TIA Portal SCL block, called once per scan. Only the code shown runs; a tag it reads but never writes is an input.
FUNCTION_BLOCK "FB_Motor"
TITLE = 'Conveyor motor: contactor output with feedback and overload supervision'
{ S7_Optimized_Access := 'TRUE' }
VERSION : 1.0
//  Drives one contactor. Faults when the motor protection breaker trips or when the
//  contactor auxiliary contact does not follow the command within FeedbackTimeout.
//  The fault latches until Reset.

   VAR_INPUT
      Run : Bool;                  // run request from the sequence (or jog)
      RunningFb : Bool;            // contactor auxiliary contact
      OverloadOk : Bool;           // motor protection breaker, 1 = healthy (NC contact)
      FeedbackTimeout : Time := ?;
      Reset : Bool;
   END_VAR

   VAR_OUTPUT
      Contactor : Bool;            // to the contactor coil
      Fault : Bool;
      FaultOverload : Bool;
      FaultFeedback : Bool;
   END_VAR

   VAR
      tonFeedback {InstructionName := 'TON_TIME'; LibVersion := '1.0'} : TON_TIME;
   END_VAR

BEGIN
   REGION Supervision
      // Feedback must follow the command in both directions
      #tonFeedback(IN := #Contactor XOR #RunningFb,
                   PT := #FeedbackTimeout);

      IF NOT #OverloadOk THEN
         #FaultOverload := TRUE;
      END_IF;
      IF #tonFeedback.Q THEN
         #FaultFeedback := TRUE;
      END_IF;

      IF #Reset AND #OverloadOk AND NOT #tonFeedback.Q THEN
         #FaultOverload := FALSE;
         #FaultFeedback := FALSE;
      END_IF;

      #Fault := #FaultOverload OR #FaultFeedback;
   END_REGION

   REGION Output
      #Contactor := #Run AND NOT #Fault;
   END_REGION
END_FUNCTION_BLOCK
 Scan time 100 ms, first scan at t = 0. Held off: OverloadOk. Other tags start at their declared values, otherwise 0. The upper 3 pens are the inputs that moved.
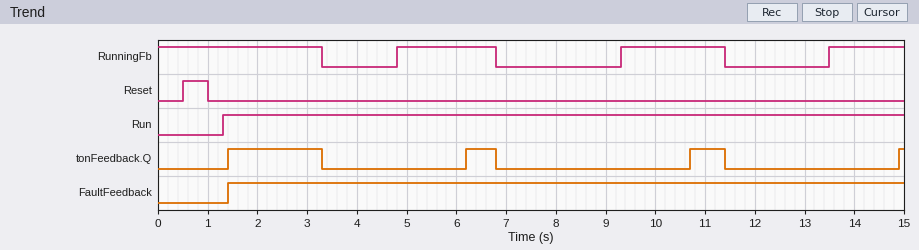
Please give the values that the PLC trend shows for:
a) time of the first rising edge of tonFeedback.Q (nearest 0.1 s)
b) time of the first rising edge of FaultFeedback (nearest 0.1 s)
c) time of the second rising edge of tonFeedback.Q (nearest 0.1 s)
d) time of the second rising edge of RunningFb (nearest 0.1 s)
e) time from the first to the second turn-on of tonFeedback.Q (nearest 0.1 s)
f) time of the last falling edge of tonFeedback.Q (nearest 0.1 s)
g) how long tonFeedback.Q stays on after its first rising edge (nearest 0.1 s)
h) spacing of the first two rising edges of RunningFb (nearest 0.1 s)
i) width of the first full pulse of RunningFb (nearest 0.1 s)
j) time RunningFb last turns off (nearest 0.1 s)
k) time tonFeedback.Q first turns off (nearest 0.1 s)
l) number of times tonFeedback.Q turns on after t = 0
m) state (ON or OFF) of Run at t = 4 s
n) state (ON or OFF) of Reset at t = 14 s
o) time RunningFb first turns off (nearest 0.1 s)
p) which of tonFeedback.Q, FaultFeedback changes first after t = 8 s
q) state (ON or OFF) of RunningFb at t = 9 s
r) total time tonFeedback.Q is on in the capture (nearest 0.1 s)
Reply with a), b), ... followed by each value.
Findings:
a) 1.4 s
b) 1.4 s
c) 6.2 s
d) 9.3 s
e) 4.8 s
f) 11.4 s
g) 1.9 s
h) 4.5 s
i) 2.0 s
j) 11.4 s
k) 3.3 s
l) 4
m) ON
n) OFF
o) 3.3 s
p) tonFeedback.Q
q) OFF
r) 3.3 s
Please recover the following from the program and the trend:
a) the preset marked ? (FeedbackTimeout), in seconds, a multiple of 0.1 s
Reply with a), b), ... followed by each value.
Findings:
a) 1.4 s
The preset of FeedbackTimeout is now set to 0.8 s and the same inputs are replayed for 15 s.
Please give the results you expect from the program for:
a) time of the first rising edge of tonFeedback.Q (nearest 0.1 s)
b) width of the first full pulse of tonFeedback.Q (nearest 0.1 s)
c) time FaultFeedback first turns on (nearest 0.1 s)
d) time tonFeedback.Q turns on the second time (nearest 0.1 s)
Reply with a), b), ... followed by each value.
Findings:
a) 0.8 s
b) 2.5 s
c) 0.8 s
d) 5.6 s
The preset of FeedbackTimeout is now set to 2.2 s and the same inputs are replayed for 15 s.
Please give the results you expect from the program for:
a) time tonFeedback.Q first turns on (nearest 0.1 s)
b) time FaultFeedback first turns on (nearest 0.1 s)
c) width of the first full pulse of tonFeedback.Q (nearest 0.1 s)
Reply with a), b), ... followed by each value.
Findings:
a) 2.2 s
b) 2.2 s
c) 1.1 s
